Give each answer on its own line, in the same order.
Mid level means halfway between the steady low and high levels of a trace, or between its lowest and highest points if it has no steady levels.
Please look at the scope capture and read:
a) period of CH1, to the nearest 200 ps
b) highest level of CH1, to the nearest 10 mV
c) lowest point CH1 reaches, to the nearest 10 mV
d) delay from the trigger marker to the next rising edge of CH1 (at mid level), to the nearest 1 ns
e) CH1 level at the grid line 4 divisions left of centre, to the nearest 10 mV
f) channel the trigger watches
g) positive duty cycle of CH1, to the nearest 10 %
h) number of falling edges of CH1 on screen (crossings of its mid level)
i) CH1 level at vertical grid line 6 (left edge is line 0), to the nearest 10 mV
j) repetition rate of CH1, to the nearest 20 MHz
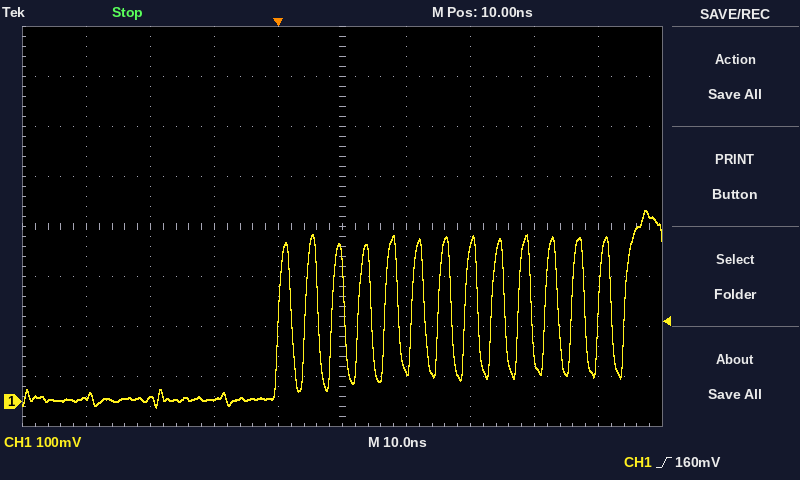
4.2 ns
380 mV
-10 mV
4 ns
10 mV
CH1
50 %
13
60 mV
240 MHz
